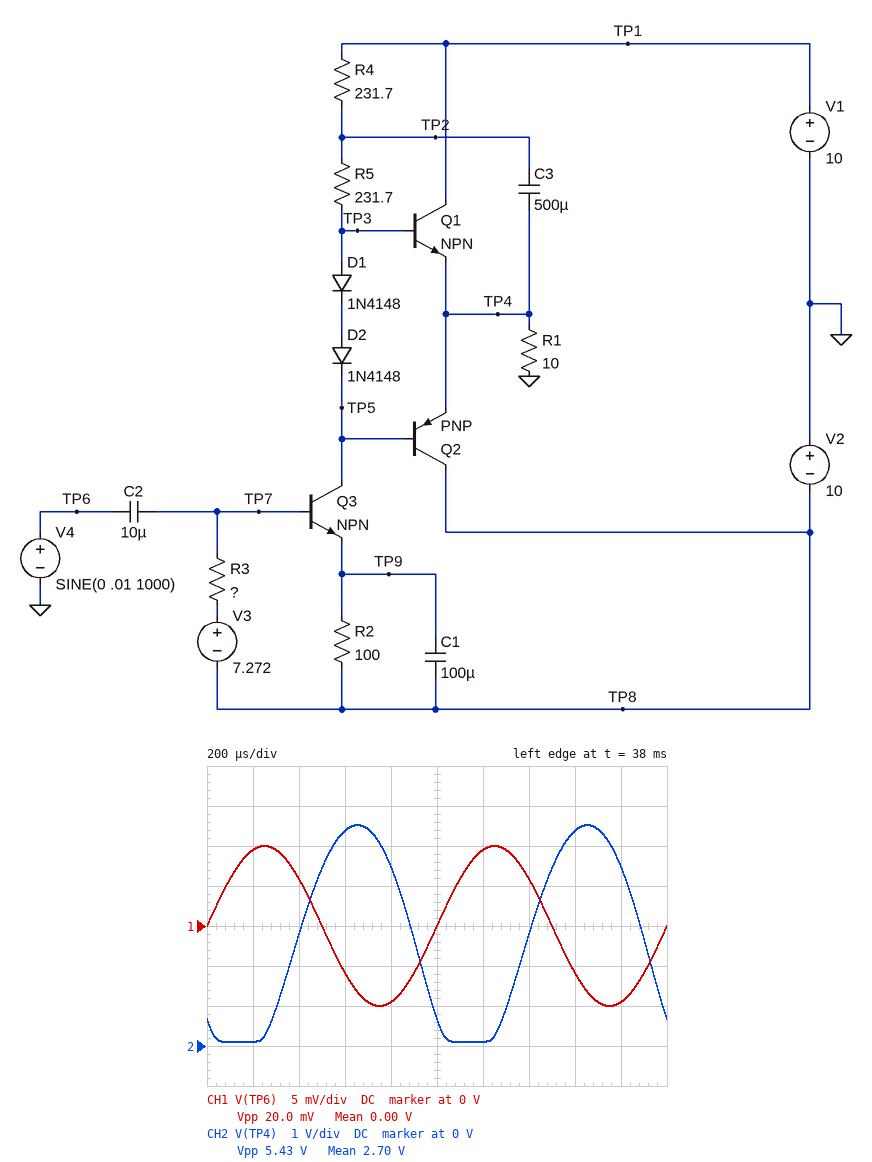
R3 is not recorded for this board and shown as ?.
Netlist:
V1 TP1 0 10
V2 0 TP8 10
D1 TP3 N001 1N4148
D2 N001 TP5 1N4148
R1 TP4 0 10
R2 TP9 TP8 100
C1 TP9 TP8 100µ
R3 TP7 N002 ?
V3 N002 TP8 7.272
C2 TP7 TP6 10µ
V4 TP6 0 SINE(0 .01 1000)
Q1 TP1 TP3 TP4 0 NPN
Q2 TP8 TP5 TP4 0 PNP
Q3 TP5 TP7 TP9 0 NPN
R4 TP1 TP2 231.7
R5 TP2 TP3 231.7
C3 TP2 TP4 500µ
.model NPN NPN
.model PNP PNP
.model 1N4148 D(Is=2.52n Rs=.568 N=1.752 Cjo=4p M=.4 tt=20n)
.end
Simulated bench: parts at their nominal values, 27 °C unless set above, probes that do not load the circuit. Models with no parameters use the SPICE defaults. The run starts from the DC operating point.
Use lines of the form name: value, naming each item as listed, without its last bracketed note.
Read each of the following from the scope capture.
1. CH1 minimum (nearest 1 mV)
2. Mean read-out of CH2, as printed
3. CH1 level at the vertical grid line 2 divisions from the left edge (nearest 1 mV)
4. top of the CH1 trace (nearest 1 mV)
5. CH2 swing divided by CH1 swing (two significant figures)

CH1 minimum: -10 mV
Mean read-out of CH2, as printed: 2.70 V
CH1 level at the vertical grid line 2 divisions from the left edge: 6 mV
top of the CH1 trace: 10 mV
CH2 swing divided by CH1 swing: 270
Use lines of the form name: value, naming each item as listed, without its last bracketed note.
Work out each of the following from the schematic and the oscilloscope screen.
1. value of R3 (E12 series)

value of R3: 47 kΩ
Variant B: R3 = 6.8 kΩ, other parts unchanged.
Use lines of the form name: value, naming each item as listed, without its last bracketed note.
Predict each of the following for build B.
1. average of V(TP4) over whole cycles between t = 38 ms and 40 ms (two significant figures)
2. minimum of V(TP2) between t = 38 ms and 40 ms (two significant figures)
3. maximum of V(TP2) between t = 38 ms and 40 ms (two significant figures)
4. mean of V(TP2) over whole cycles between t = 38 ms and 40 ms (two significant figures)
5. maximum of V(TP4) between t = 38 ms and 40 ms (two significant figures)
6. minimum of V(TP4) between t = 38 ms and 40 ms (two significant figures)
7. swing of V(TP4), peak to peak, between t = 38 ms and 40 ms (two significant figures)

average of V(TP4) over whole cycles between t = 38 ms and 40 ms: -3.6 V
minimum of V(TP2) between t = 38 ms and 40 ms: 2.0 V
maximum of V(TP2) between t = 38 ms and 40 ms: 7.2 V
mean of V(TP2) over whole cycles between t = 38 ms and 40 ms: 3.9 V
maximum of V(TP4) between t = 38 ms and 40 ms: -320 mV
minimum of V(TP4) between t = 38 ms and 40 ms: -5.5 V
swing of V(TP4), peak to peak, between t = 38 ms and 40 ms: 5.2 V
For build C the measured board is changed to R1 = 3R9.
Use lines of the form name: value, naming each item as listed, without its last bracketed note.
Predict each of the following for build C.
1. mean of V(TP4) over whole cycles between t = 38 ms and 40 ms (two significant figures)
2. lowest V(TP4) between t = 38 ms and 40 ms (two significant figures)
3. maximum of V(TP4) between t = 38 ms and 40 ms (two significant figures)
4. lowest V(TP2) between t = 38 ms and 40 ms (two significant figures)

mean of V(TP4) over whole cycles between t = 38 ms and 40 ms: 1.8 V
lowest V(TP4) between t = 38 ms and 40 ms: 420 mV
maximum of V(TP4) between t = 38 ms and 40 ms: 3.0 V
lowest V(TP2) between t = 38 ms and 40 ms: 5.0 V
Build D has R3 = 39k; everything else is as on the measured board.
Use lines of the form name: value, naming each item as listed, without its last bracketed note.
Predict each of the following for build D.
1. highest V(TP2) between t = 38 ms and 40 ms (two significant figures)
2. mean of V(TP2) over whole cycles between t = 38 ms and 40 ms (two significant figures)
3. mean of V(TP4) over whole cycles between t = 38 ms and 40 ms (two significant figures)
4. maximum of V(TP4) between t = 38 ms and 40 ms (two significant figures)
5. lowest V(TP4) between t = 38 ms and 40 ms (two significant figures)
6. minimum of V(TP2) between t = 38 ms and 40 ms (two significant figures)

highest V(TP2) between t = 38 ms and 40 ms: 9.5 V
mean of V(TP2) over whole cycles between t = 38 ms and 40 ms: 6.5 V
mean of V(TP4) over whole cycles between t = 38 ms and 40 ms: 2.2 V
maximum of V(TP4) between t = 38 ms and 40 ms: 5.1 V
lowest V(TP4) between t = 38 ms and 40 ms: -540 mV
minimum of V(TP2) between t = 38 ms and 40 ms: 3.8 V
